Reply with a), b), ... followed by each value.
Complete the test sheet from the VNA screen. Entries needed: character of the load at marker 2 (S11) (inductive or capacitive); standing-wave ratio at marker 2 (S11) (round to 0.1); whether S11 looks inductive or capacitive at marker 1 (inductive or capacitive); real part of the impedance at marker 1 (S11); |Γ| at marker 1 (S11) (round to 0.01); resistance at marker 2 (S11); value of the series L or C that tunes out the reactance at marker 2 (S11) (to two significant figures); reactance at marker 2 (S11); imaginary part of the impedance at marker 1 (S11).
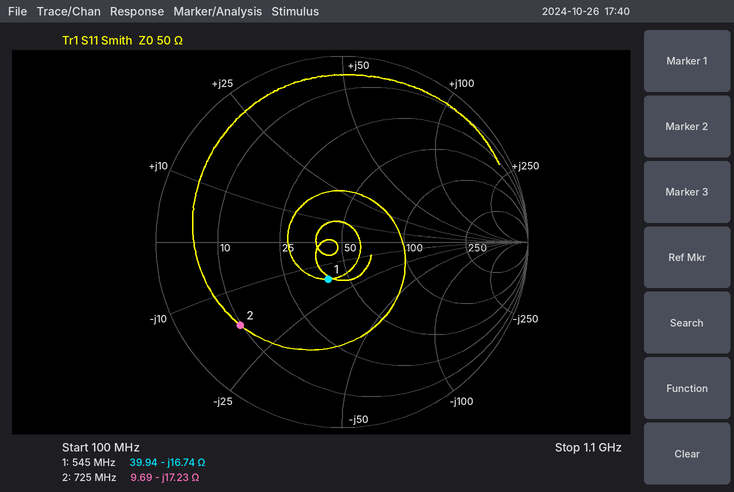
a) capacitive
b) 5.8
c) capacitive
d) 39.94 Ω
e) 0.21
f) 9.69 Ω
g) 3.8 nH
h) -17.23 Ω
i) -16.74 Ω
